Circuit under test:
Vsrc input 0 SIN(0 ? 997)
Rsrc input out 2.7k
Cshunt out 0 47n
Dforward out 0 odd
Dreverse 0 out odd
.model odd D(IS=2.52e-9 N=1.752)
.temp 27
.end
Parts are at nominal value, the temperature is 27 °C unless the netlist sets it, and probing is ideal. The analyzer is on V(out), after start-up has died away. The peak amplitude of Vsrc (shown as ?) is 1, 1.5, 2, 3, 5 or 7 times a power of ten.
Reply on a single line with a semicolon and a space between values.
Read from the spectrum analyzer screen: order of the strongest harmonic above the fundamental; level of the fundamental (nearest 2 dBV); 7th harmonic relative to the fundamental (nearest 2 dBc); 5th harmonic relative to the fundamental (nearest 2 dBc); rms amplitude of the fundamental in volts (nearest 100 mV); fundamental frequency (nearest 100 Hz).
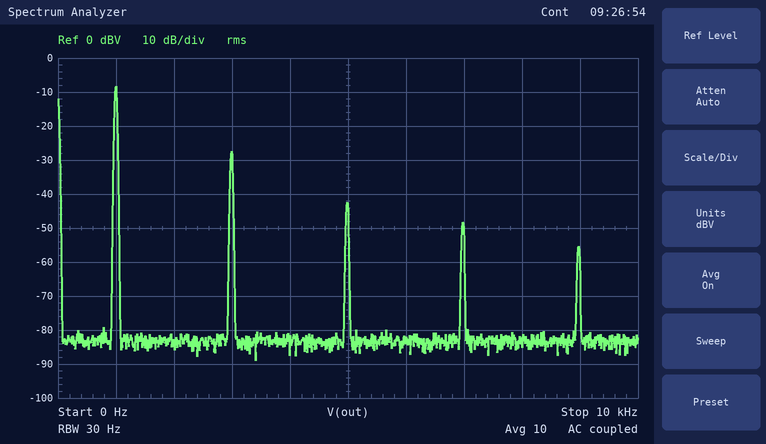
3; -8 dBV; -40 dBc; -34 dBc; 400 mV; 1.0 kHz
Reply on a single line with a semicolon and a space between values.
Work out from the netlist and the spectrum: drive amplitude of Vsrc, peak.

1 V
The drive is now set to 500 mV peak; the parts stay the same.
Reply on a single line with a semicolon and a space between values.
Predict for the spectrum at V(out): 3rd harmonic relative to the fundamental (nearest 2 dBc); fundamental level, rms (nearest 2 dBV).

-40 dBc; -12 dBV
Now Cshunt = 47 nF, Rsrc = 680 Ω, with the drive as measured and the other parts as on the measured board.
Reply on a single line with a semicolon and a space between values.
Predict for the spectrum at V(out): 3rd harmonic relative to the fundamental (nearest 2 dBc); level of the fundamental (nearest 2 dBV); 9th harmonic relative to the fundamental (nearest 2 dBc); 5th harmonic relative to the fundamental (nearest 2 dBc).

-16 dBc; -6 dBV; -42 dBc; -32 dBc
